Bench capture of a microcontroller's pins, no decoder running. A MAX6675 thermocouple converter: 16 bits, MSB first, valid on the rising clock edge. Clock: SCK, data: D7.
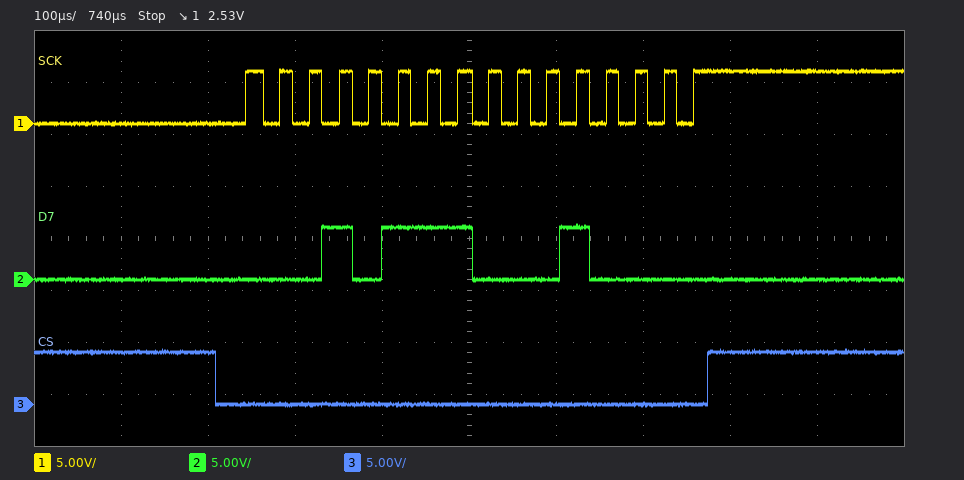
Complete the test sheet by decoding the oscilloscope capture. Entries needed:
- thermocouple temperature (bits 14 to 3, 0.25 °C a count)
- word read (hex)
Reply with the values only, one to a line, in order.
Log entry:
184.50 °C
0x1710
